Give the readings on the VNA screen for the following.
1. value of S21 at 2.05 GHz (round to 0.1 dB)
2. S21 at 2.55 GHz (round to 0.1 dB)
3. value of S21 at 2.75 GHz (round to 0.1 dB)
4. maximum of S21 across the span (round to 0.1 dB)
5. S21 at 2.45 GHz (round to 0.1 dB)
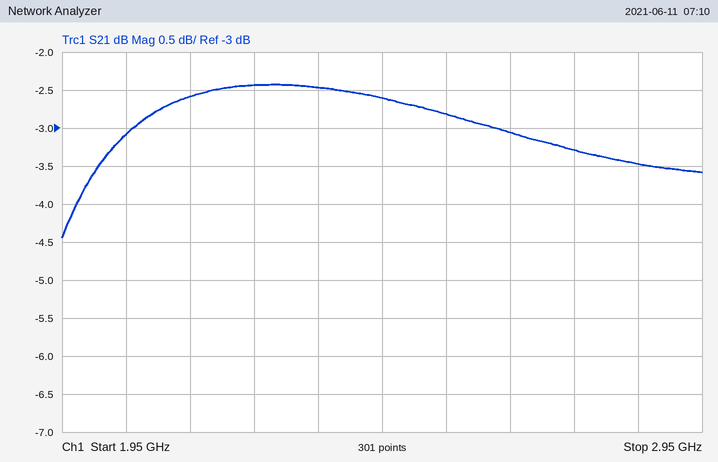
-3.1 dB
-2.8 dB
-3.3 dB
-2.4 dB
-2.6 dB
